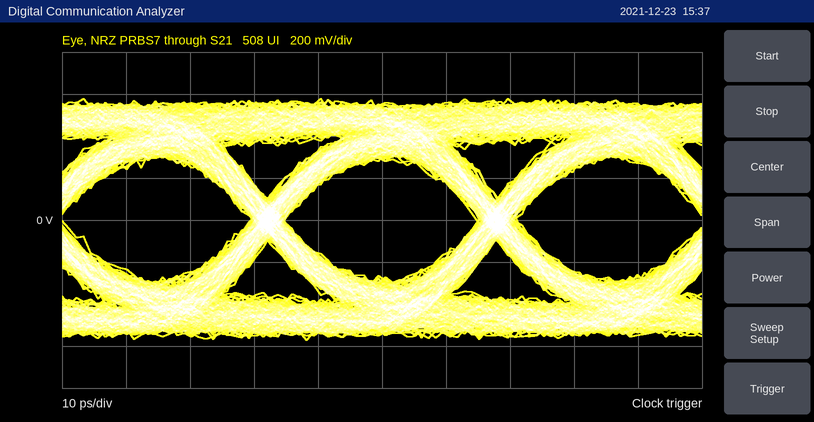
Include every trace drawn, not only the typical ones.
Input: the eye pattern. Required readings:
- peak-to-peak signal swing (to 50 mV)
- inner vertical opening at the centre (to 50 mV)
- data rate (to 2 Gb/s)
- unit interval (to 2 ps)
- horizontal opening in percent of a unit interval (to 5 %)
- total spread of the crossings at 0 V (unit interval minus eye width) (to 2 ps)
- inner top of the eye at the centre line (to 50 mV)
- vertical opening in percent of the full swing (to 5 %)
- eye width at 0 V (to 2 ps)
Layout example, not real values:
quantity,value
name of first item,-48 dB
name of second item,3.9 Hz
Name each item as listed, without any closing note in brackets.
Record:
quantity,value
peak-to-peak signal swing,1.15 V
inner vertical opening at the centre,550 mV
data rate,28 Gb/s
unit interval,36 ps
horizontal opening in percent of a unit interval,85 %
total spread of the crossings at 0 V (unit interval minus eye width),6 ps
inner top of the eye at the centre line,300 mV
vertical opening in percent of the full swing,50 %
eye width at 0 V,30 ps
